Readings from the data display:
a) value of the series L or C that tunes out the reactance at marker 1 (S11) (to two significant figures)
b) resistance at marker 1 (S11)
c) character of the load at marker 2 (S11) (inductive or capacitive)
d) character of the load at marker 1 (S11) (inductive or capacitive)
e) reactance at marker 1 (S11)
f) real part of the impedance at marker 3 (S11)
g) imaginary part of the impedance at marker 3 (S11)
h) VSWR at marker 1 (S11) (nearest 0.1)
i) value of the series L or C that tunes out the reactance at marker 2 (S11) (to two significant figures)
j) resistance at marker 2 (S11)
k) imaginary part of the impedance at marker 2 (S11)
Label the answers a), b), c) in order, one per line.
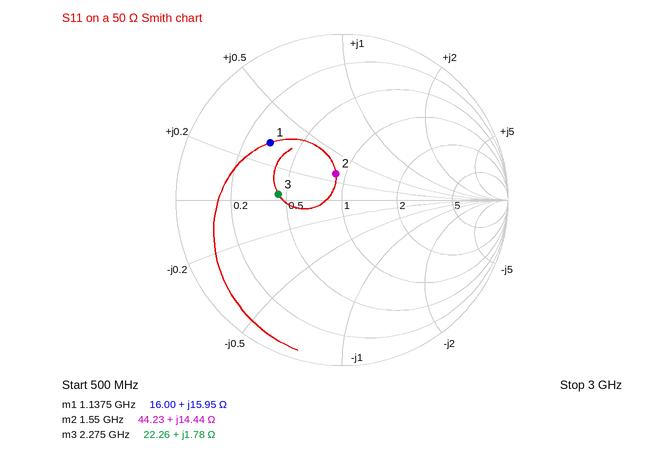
a) 8.8 pF
b) 16.00 Ω
c) inductive
d) inductive
e) +15.95 Ω
f) 22.26 Ω
g) +1.78 Ω
h) 3.5
i) 7.1 pF
j) 44.23 Ω
k) +14.44 Ω
